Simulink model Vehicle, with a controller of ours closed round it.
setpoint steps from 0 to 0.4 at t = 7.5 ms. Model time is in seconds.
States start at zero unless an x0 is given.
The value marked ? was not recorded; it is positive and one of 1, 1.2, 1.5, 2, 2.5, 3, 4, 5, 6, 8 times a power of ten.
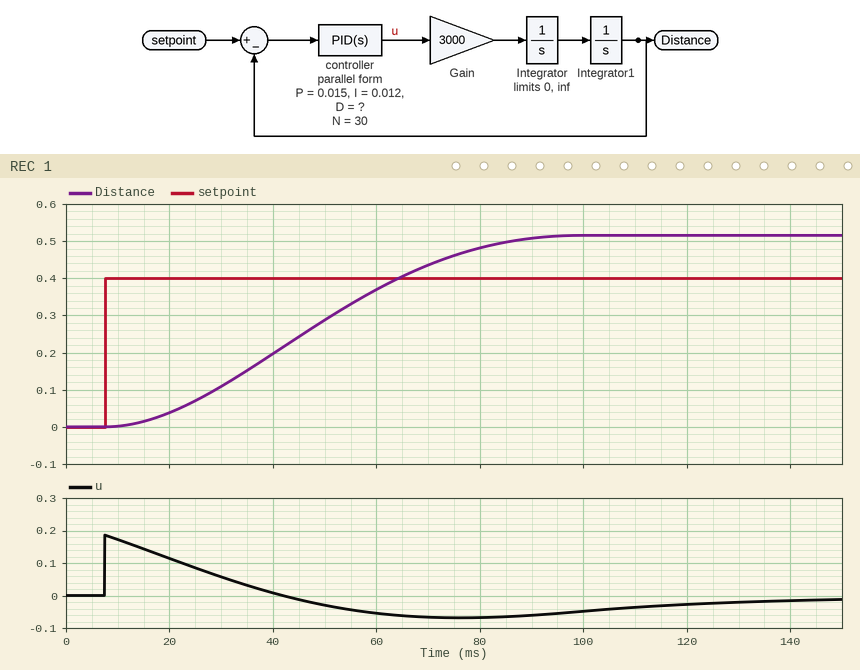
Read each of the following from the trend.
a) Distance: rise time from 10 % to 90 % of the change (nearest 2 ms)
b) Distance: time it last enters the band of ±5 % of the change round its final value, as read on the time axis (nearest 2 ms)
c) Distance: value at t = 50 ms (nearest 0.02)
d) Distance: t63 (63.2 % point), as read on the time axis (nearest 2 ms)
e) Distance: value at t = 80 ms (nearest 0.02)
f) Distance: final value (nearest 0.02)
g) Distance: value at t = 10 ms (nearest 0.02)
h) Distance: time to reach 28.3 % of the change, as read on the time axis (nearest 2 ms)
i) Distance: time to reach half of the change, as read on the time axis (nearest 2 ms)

54 ms
82 ms
0.28
54 ms
0.48
0.52
0.00
34 ms
46 ms
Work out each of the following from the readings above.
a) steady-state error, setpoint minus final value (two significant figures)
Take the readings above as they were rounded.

-0.12
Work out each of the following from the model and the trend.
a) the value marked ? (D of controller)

0.015
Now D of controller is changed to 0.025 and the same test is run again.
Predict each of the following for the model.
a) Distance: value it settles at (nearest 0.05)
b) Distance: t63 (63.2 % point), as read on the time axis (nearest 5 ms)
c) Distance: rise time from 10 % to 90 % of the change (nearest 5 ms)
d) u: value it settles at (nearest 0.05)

0.55
45 ms
40 ms
0.00
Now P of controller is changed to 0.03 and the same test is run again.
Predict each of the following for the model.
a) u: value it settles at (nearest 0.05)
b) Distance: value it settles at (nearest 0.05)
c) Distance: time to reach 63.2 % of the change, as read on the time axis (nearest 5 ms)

0.00
0.55
55 ms
